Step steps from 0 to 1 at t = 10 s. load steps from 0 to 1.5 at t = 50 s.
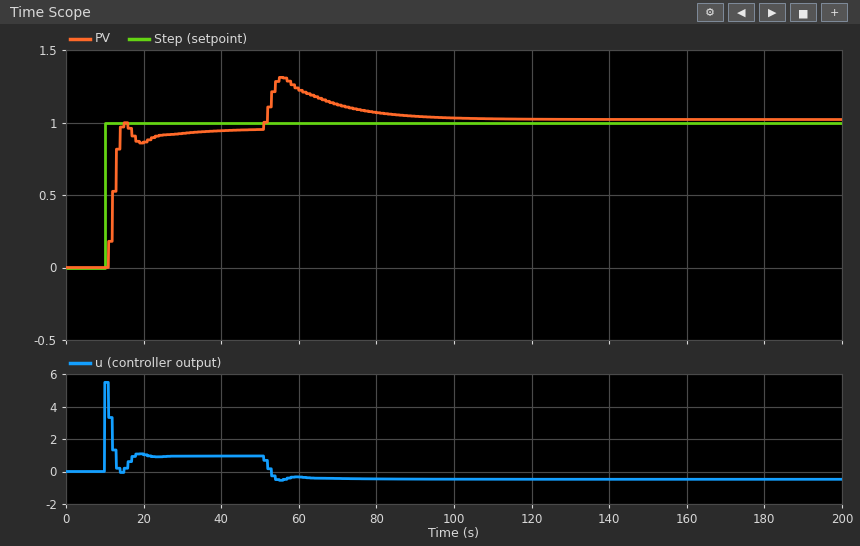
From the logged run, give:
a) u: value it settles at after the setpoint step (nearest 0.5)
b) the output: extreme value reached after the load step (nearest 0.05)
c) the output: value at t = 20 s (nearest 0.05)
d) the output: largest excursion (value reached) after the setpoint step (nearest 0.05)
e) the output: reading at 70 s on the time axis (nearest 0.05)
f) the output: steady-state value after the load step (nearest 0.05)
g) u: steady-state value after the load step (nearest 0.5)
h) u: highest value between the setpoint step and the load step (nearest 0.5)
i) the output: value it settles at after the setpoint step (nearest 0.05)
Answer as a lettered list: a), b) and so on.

a) 1.0
b) 1.30
c) 0.85
d) 1.00
e) 1.10
f) 1.00
g) -0.5
h) 5.5
i) 0.95
